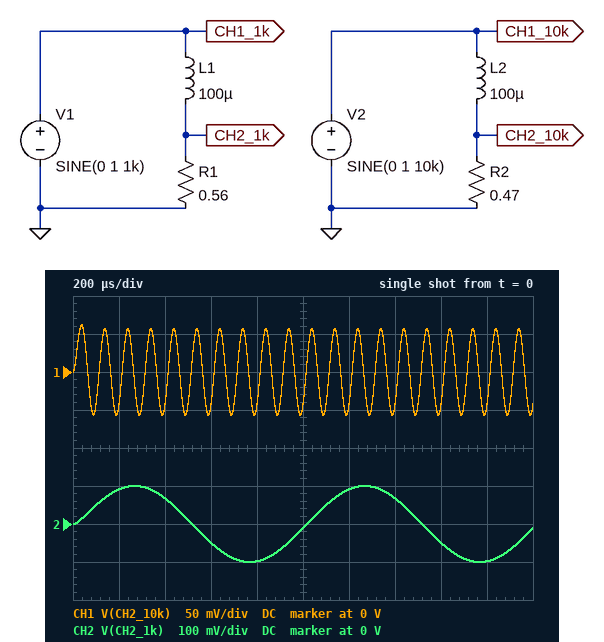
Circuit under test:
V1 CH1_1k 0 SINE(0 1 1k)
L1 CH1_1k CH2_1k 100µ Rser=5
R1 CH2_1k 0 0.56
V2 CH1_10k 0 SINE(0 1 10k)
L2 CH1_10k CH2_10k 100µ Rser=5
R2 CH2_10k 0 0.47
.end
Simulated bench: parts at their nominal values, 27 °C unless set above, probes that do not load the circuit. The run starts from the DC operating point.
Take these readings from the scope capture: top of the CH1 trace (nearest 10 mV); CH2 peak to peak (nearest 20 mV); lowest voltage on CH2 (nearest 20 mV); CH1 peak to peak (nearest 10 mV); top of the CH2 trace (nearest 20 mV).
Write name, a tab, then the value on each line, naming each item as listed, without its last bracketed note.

top of the CH1 trace	60 mV
CH2 peak to peak	200 mV
lowest voltage on CH2	-100 mV
CH1 peak to peak	120 mV
top of the CH2 trace	100 mV
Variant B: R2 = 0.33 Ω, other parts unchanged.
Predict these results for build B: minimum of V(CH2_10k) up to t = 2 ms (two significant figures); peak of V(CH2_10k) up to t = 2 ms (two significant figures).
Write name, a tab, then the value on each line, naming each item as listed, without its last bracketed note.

minimum of V(CH2_10k) up to t = 2 ms	-40 mV
peak of V(CH2_10k) up to t = 2 ms	44 mV
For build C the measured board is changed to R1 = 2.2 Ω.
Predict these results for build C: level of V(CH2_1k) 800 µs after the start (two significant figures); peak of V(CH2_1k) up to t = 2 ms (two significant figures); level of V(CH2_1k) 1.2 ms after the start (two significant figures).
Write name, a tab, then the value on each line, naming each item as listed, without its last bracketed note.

level of V(CH2_1k) 800 µs after the start	-300 mV
peak of V(CH2_1k) up to t = 2 ms	300 mV
level of V(CH2_1k) 1.2 ms after the start	280 mV
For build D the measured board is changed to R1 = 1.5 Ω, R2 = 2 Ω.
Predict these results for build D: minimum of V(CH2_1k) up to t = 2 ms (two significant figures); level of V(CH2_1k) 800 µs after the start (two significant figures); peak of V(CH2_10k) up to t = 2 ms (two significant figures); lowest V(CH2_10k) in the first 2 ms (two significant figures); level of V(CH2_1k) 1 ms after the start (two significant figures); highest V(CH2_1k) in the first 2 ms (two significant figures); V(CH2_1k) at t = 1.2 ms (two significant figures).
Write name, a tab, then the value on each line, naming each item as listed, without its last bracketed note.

minimum of V(CH2_1k) up to t = 2 ms	-230 mV
level of V(CH2_1k) 800 µs after the start	-220 mV
peak of V(CH2_10k) up to t = 2 ms	220 mV
lowest V(CH2_10k) in the first 2 ms	-210 mV
level of V(CH2_1k) 1 ms after the start	-22 mV
highest V(CH2_1k) in the first 2 ms	230 mV
V(CH2_1k) at t = 1.2 ms	210 mV
